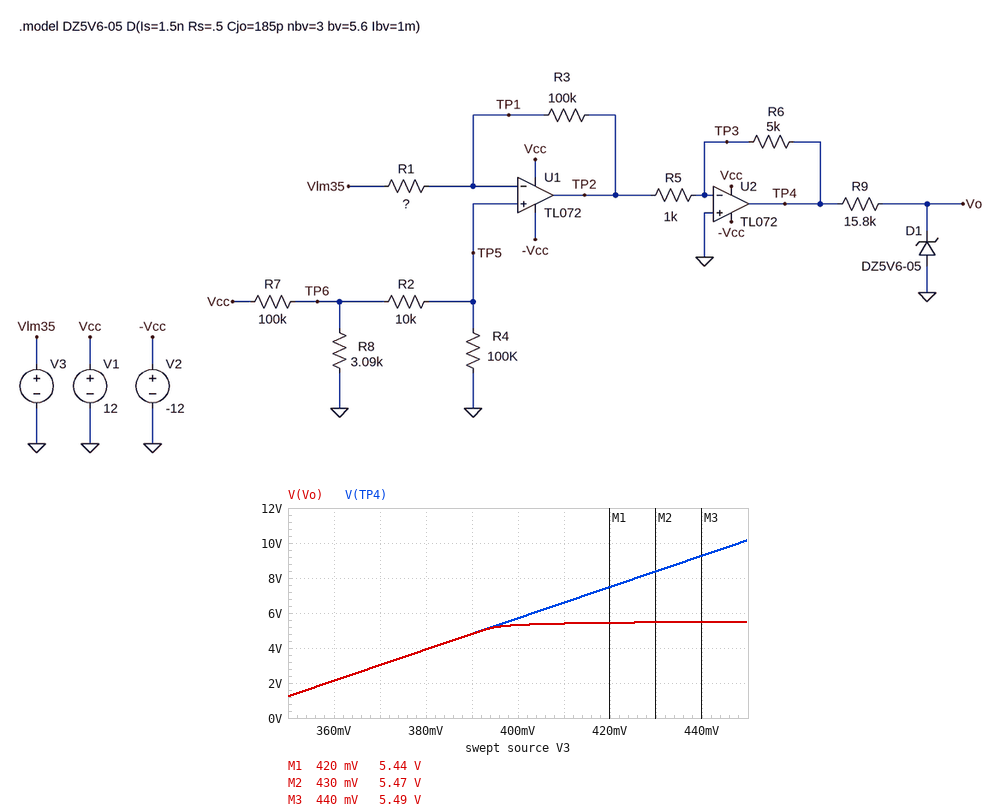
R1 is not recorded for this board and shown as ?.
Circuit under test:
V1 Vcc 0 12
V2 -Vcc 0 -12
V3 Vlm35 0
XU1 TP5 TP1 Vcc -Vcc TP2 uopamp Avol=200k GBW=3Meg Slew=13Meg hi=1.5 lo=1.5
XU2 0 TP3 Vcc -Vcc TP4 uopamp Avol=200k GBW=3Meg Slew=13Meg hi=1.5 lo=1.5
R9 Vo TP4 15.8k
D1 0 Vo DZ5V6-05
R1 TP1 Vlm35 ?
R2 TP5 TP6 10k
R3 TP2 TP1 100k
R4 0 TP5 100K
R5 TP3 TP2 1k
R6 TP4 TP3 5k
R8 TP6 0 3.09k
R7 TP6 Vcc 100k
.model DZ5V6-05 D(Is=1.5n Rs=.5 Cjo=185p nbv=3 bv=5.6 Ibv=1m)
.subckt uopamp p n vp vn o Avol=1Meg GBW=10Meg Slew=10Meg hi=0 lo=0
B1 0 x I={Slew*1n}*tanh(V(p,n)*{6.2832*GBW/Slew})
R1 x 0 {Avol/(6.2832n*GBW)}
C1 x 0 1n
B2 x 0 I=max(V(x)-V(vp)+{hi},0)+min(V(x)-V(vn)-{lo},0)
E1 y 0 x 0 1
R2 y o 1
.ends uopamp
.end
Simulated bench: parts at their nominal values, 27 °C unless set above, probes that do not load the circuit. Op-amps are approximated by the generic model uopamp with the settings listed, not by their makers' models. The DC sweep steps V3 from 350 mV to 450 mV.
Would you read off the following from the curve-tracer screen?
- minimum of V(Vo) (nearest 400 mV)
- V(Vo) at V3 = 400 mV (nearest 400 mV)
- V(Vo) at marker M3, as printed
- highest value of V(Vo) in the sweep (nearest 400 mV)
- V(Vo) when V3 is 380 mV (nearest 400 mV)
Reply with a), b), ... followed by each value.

a) 1.2 V
b) 5.2 V
c) 5.49 V
d) 5.6 V
e) 4.0 V
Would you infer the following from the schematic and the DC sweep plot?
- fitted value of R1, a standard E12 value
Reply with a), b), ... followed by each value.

a) 5.6 kΩ
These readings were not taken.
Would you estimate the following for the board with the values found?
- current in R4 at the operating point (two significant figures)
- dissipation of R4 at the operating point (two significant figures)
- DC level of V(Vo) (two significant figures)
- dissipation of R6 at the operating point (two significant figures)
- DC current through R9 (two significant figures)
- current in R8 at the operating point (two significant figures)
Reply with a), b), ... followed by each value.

a) 3.2 µA
b) 1.0 µW
c) -340 mV
d) 38 mW
e) 640 µA
f) 110 µA
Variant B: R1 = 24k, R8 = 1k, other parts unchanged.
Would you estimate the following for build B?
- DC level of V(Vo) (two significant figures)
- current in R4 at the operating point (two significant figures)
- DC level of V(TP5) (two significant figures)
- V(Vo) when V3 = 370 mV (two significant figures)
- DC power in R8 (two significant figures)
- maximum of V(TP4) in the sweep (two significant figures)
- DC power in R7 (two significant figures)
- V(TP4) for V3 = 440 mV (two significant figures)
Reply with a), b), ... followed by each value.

a) -300 mV
b) 1.1 µA
c) 110 mV
d) 4.9 V
e) 14 µW
f) 6.6 V
g) 1.4 mW
h) 6.4 V
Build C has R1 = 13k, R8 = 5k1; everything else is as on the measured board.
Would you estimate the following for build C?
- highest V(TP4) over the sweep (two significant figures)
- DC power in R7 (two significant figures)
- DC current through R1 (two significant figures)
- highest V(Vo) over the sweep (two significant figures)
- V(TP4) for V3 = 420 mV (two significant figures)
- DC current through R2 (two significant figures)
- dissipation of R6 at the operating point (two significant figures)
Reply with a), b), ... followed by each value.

a) -4.7 V
b) 1.3 mW
c) 39 µA
d) -310 mV
e) -5.9 V
f) 5.1 µA
g) 31 mW
